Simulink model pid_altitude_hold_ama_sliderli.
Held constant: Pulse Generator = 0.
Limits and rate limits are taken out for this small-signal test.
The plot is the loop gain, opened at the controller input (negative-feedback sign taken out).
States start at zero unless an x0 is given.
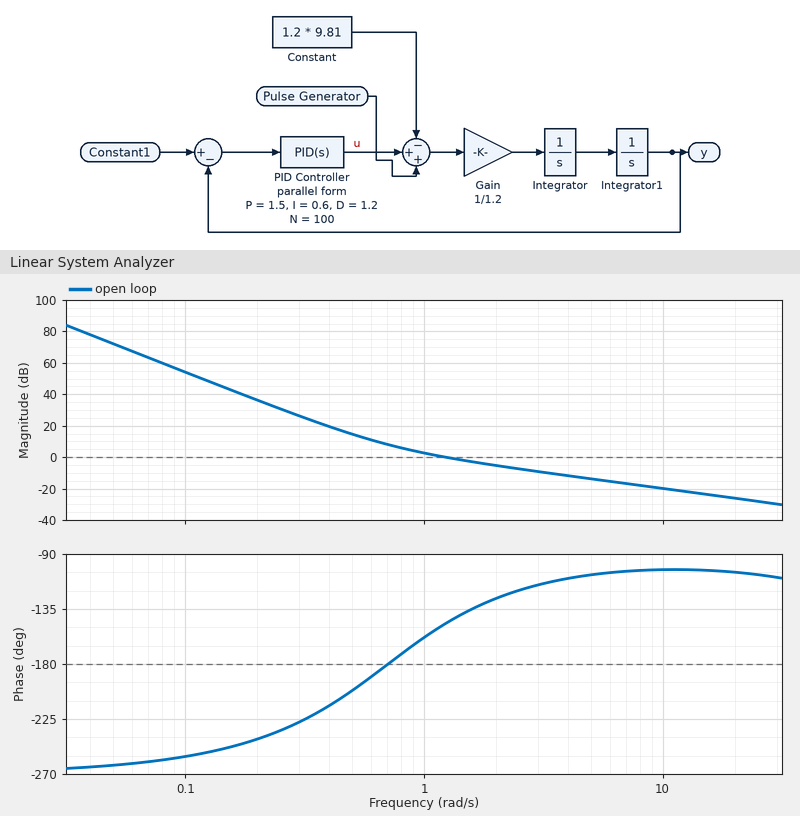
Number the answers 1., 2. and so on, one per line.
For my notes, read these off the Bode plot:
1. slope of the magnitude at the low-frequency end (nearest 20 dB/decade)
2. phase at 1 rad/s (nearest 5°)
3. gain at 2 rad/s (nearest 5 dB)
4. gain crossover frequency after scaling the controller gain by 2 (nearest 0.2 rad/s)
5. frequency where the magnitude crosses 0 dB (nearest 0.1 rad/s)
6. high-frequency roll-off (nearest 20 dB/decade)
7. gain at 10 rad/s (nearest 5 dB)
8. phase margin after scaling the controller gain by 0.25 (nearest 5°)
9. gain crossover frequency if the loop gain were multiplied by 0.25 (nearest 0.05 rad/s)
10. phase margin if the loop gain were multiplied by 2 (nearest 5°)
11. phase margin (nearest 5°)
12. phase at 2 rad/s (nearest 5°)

1. -60 dB/decade
2. -160°
3. -5 dB
4. 2.2 rad/s
5. 1.2 rad/s
6. -20 dB/decade
7. -20 dB
8. -15°
9. 0.55 rad/s
10. 55°
11. 35°
12. -125°
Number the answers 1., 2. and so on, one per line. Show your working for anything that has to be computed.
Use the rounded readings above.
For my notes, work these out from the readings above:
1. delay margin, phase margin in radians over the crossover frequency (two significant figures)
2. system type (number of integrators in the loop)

1. 35 × π / 180 / 1.2 = 0.51 s
2. 3
